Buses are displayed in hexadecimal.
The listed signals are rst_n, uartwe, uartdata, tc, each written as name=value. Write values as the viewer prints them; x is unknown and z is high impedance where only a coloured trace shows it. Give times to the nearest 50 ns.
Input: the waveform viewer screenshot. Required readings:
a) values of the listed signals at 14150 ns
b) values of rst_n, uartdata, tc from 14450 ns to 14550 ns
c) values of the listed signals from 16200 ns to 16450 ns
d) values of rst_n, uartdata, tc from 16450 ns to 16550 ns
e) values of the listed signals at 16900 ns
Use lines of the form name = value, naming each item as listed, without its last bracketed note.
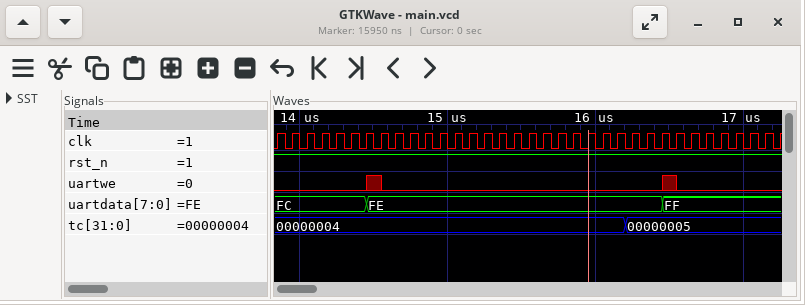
values of the listed signals at 14150 ns = rst_n=1, uartwe=0, uartdata=FC, tc=00000004
values of rst_n, uartdata, tc from 14450 ns to 14550 ns = rst_n=1, uartdata=FE, tc=00000004
values of the listed signals from 16200 ns to 16450 ns = rst_n=1, uartwe=0, uartdata=FE, tc=00000005
values of rst_n, uartdata, tc from 16450 ns to 16550 ns = rst_n=1, uartdata=FF, tc=00000005
values of the listed signals at 16900 ns = rst_n=1, uartwe=0, uartdata=FF, tc=00000005
